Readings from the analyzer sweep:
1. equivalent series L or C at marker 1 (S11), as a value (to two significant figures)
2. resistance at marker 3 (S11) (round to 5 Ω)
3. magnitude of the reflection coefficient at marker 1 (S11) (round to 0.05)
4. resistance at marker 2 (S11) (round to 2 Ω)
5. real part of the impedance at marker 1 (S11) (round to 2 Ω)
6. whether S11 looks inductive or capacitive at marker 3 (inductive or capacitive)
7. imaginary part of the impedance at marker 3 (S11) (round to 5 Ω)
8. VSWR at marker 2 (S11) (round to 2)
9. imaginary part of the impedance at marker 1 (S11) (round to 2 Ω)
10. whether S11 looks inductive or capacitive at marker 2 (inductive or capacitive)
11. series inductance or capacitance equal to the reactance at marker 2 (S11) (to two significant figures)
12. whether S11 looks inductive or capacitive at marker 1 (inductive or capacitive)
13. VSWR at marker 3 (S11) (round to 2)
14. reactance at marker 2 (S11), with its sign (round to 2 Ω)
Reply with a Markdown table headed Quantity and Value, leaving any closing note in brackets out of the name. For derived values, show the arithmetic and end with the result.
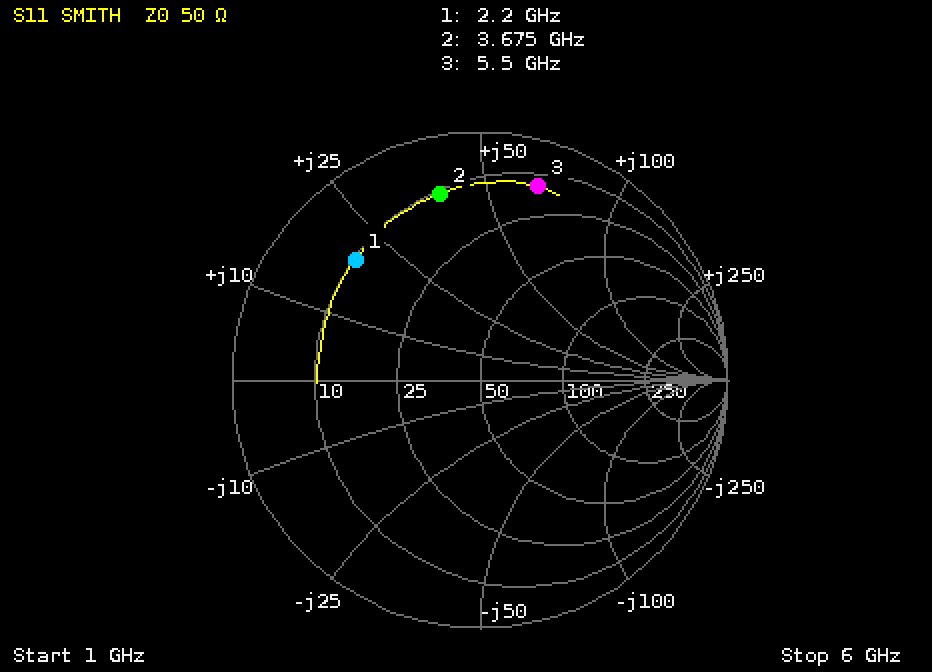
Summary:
| Quantity | Value |
|---|---|
| equivalent series L or C at marker 1 (S11), as a value | L = 20 Ω/(2π × 2.2 GHz) ≈ 1.4 nH |
| resistance at marker 3 (S11) | 15 Ω |
| magnitude of the reflection coefficient at marker 1 (S11) | 0.70 |
| resistance at marker 2 (S11) | 10 Ω |
| real part of the impedance at marker 1 (S11) | 10 Ω |
| whether S11 looks inductive or capacitive at marker 3 | inductive |
| imaginary part of the impedance at marker 3 (S11) | +65 Ω |
| VSWR at marker 2 (S11) | 8 |
| imaginary part of the impedance at marker 1 (S11) | +20 Ω |
| whether S11 looks inductive or capacitive at marker 2 | inductive |
| series inductance or capacitance equal to the reactance at marker 2 (S11) | L = 40 Ω/(2π × 3.675 GHz) ≈ 1.7 nH |
| whether S11 looks inductive or capacitive at marker 1 | inductive |
| VSWR at marker 3 (S11) | 10 |
| reactance at marker 2 (S11), with its sign | +40 Ω |
